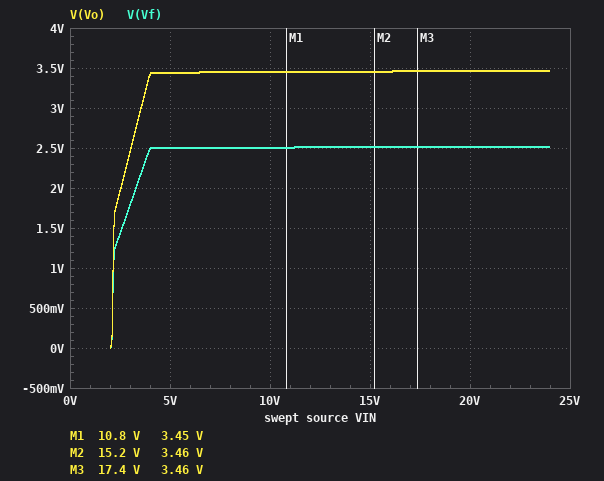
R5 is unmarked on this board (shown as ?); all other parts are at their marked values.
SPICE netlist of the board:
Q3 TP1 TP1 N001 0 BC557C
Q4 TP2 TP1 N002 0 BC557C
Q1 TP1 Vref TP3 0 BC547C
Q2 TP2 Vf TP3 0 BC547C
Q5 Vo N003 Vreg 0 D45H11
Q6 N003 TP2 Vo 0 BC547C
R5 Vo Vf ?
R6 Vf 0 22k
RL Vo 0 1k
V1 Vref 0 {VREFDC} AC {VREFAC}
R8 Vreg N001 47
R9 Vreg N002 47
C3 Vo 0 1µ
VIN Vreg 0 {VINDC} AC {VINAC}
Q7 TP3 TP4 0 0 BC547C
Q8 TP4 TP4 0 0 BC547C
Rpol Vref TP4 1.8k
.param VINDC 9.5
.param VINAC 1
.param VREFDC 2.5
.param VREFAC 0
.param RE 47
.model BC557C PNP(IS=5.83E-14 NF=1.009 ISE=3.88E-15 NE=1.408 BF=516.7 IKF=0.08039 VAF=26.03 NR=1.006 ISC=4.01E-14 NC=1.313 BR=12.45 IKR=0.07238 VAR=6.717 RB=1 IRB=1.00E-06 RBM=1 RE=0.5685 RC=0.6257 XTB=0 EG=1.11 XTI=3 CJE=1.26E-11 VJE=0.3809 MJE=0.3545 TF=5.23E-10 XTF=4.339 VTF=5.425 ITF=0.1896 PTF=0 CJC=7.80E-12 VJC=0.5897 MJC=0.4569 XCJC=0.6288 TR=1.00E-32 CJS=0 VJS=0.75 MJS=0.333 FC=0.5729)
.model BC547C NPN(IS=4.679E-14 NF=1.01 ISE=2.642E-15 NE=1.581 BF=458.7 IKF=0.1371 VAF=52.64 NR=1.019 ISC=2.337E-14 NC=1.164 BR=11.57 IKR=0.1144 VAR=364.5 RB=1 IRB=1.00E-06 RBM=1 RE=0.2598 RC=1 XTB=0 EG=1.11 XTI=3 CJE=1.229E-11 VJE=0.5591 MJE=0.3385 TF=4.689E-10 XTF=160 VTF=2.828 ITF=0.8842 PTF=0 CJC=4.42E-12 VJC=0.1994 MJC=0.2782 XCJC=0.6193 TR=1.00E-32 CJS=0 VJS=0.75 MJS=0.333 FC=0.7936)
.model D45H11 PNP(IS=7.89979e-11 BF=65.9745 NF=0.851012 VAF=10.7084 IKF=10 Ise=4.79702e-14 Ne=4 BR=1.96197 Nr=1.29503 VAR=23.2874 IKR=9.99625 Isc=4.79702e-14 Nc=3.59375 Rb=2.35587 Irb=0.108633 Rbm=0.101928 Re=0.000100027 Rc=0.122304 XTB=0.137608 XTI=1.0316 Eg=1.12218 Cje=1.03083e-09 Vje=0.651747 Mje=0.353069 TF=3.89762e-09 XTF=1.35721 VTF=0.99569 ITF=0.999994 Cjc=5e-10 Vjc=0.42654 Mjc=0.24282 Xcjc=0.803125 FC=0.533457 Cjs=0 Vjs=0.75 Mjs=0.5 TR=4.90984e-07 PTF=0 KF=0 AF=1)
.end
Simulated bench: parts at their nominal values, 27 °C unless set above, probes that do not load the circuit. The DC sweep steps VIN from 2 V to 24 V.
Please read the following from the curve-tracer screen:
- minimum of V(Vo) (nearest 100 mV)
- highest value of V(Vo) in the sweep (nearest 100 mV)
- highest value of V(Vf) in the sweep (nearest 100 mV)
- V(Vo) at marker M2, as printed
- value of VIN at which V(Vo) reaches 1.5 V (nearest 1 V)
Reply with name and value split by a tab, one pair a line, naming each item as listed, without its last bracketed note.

minimum of V(Vo)	0 V
highest value of V(Vo) in the sweep	3.5 V
highest value of V(Vf) in the sweep	2.5 V
V(Vo) at marker M2, as printed	3.46 V
value of VIN at which V(Vo) reaches 1.5 V	2 V
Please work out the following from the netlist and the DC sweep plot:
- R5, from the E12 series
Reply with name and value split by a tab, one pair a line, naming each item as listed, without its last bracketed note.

R5, from the E12 series	8.2 kΩ
